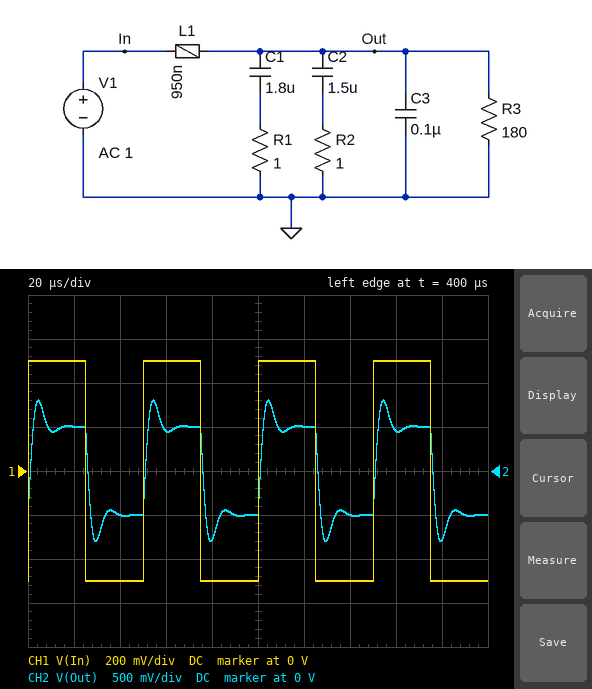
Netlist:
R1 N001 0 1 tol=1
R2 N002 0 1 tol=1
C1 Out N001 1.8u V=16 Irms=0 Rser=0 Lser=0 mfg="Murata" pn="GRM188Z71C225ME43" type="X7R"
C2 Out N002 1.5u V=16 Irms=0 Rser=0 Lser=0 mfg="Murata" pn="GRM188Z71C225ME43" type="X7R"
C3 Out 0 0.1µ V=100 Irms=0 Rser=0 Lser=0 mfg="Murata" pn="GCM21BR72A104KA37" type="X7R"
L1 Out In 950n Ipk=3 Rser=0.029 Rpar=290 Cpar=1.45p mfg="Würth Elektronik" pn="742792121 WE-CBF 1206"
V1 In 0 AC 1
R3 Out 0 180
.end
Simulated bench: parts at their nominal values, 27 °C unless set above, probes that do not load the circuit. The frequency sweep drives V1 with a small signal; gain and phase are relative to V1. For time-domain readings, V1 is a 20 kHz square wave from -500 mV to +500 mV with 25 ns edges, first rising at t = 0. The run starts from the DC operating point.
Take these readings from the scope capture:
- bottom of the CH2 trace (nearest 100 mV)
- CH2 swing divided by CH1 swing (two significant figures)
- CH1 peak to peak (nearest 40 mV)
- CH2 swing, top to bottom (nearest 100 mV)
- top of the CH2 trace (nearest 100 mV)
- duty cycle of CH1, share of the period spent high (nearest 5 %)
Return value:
-800 mV
1.6
1.00 V
1.6 V
800 mV
50 %
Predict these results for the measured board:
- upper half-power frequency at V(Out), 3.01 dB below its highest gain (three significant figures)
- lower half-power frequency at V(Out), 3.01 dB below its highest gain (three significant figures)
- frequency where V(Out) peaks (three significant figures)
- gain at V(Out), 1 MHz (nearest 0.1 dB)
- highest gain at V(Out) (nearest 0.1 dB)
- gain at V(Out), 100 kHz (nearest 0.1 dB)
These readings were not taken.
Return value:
121 kHz
18.8 kHz
76.9 kHz
-21.9 dB
3.4 dB
2.3 dB
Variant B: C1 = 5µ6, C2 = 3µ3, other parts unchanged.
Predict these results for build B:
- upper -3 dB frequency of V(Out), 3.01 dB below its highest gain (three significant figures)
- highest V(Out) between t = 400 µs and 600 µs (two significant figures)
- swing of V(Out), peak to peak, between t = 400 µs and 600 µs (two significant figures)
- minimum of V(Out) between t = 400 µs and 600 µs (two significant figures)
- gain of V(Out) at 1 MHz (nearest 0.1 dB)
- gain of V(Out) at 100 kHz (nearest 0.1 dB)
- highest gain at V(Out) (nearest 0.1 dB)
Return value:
96.4 kHz
660 mV
1.3 V
-660 mV
-21.9 dB
-1.8 dB
1.5 dB
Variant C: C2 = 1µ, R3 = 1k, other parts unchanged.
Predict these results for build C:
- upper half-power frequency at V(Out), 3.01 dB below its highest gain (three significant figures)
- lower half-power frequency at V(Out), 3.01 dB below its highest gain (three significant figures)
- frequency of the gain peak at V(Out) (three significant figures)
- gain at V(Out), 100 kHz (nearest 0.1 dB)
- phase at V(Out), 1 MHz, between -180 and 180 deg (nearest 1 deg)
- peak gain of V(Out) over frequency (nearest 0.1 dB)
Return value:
132 kHz
27.7 kHz
86.3 kHz
3.3 dB
-108 deg
3.7 dB
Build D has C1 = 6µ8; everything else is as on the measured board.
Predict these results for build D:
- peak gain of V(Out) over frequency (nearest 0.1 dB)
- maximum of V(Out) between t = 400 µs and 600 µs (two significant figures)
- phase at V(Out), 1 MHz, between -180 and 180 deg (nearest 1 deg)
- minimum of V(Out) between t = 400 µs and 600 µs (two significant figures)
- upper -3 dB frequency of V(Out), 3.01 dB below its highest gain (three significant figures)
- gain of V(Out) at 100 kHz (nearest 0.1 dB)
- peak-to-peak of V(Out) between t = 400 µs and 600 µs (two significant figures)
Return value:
1.4 dB
660 mV
-105 deg
-660 mV
118 kHz
-0.4 dB
1.3 V
